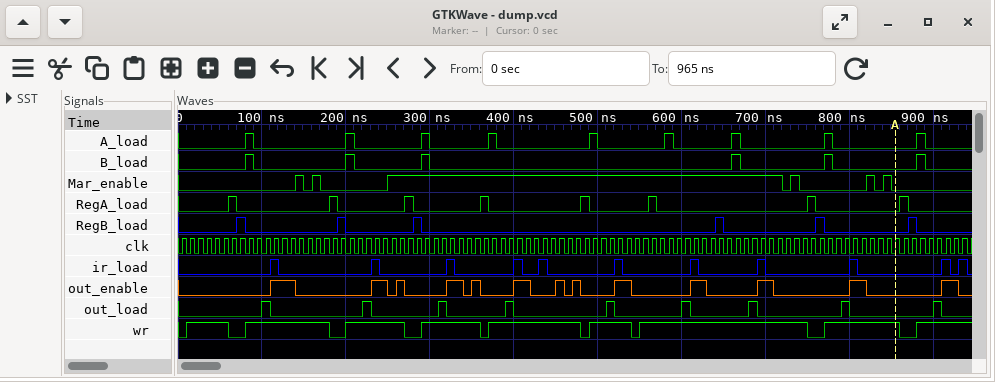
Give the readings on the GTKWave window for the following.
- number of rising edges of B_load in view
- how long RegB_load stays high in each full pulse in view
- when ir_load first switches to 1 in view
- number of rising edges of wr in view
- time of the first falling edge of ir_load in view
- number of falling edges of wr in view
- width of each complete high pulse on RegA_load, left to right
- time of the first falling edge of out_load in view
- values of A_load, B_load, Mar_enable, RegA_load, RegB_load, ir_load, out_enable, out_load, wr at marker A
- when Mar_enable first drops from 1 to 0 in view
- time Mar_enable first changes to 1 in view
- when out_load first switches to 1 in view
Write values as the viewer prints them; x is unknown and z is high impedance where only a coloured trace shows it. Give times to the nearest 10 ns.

6
10 ns, 10 ns, 10 ns, 10 ns, 10 ns, 10 ns
110 ns
9
120 ns
8
10 ns, 10 ns, 10 ns, 10 ns, 10 ns, 10 ns, 10 ns, 10 ns
110 ns
A_load=0, B_load=0, Mar_enable=0, RegA_load=0, RegB_load=0, ir_load=0, out_enable=0, out_load=0, wr=1
150 ns
140 ns
100 ns
